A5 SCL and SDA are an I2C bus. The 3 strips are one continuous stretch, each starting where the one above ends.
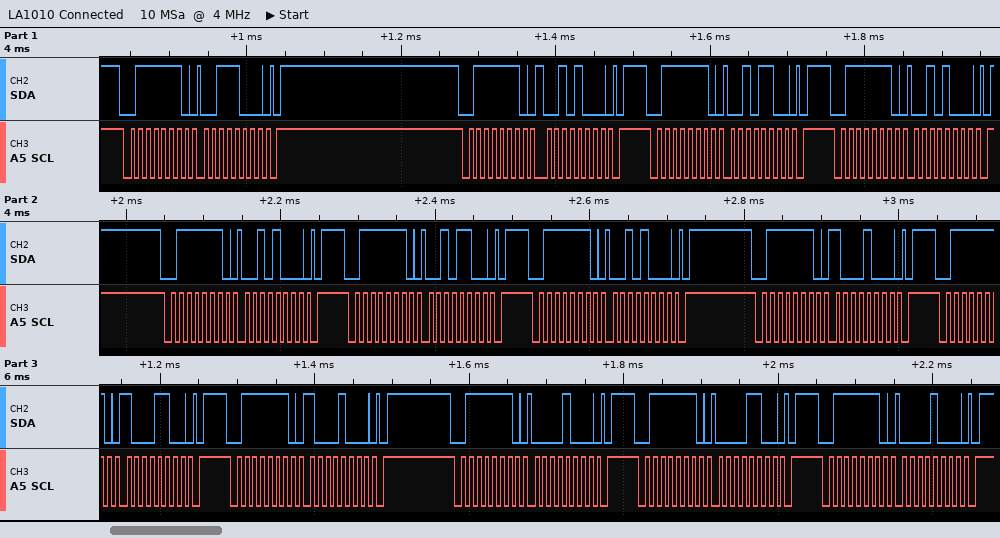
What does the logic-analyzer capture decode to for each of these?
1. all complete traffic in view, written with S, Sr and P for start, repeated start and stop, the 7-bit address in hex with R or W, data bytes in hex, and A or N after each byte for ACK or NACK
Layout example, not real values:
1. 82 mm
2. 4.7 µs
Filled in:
1. S 3FW A 38 A P S 3FW A 28 A P S 3FW A 2C A P S 3FW A 28 A P S 3FW A 28 A P S 3FW A 2C A P S 3FW A 28 A P S 3FW A 88 A P S 3FW A 8C A P S 3FW A 88 A P S 3FW A 08 A P S 3FW A 0C A P S 3FW A 08 A P
